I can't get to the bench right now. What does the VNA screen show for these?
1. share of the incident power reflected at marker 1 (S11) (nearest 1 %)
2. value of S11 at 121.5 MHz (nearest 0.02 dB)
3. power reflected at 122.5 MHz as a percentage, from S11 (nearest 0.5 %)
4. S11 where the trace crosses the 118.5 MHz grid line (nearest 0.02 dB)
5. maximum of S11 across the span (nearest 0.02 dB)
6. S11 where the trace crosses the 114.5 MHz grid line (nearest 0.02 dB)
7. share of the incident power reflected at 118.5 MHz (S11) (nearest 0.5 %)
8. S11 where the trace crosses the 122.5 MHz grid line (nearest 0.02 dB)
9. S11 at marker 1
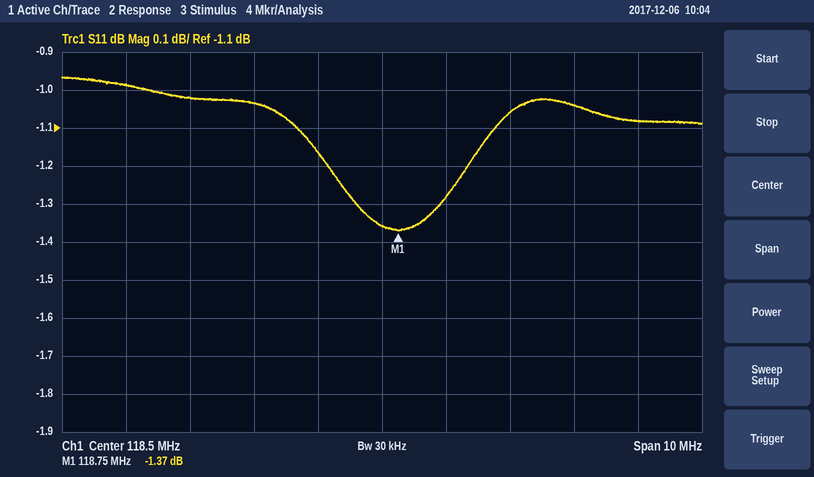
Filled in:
73 %
-1.04 dB
78.0 %
-1.36 dB
-0.96 dB
-0.98 dB
73.0 %
-1.08 dB
-1.37 dB
